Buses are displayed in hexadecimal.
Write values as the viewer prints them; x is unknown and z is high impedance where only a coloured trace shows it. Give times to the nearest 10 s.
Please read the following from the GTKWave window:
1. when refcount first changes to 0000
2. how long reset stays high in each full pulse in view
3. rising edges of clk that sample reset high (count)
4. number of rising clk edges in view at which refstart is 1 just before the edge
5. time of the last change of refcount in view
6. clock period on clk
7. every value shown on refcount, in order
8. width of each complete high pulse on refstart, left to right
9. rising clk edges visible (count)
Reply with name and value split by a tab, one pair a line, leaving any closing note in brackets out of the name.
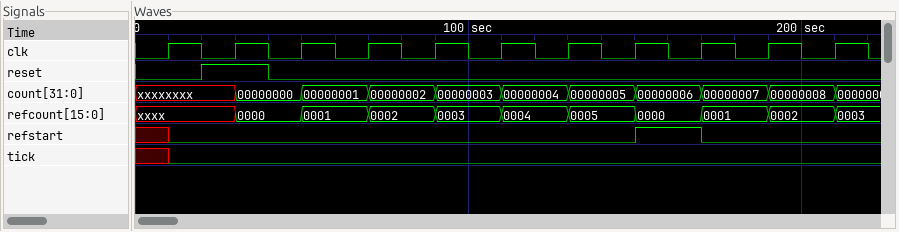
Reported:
when refcount first changes to 0000	30 s
how long reset stays high in each full pulse in view	20 s
rising edges of clk that sample reset high	1
number of rising clk edges in view at which refstart is 1 just before the edge	1
time of the last change of refcount in view	210 s
clock period on clk	20 s
every value shown on refcount, in order	xxxx, 0000, 0001, 0002, 0003, 0004, 0005, 0000, 0001, 0002, 0003
width of each complete high pulse on refstart, left to right	20 s
rising clk edges visible	11
